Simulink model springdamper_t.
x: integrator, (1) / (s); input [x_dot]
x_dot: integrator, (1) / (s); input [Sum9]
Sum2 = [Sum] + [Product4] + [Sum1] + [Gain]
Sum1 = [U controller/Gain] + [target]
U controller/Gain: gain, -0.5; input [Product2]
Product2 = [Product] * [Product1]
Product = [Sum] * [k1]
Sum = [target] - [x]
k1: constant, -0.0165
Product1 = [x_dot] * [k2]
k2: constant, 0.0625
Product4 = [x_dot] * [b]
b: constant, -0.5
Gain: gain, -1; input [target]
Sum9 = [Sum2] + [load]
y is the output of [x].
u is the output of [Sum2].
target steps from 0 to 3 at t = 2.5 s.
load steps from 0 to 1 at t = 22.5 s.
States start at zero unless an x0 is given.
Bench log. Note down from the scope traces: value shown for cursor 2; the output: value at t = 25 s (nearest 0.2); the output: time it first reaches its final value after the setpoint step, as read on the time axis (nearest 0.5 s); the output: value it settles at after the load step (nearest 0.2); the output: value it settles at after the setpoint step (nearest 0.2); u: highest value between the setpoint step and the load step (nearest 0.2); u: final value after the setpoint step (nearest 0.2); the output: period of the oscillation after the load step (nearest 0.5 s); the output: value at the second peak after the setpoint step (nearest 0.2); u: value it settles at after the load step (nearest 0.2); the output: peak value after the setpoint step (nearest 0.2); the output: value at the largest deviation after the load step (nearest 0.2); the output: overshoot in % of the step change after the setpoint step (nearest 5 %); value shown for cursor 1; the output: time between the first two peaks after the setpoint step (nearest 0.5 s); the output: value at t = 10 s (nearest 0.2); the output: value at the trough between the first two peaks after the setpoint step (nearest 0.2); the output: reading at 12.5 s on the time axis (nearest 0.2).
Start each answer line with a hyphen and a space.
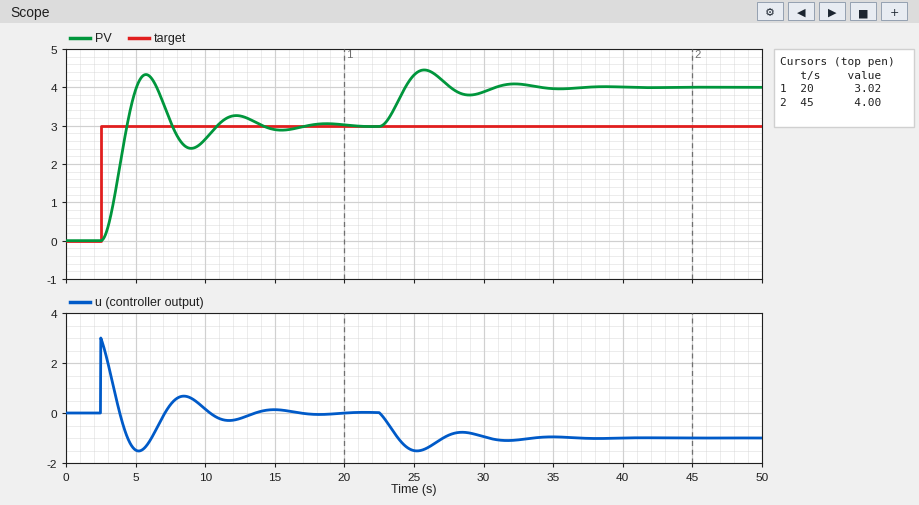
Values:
- 4.00
- 4.4
- 4.5 s
- 4.0
- 3.0
- 3.0
- 0.0
- 6.5 s
- 3.2
- -1.0
- 4.4
- 4.4
- 45 %
- 3.02
- 6.5 s
- 2.6
- 2.4
- 3.2
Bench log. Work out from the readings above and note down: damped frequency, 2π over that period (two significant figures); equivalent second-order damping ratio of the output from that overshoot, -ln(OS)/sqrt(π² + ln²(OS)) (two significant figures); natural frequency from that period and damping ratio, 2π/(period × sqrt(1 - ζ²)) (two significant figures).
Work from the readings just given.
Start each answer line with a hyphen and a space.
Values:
- 0.97 rad/s
- 0.25
- 1.00 rad/s
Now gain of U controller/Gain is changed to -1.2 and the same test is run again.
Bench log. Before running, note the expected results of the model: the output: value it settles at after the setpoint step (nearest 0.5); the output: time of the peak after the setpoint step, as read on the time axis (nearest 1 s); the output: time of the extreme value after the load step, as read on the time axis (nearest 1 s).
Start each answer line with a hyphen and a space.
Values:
- 3.0
- 6 s
- 26 s
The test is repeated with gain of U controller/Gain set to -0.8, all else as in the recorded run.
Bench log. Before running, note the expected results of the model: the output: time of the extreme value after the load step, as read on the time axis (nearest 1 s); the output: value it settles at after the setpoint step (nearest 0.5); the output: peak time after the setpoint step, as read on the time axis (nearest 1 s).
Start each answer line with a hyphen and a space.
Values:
- 26 s
- 3.0
- 6 s
